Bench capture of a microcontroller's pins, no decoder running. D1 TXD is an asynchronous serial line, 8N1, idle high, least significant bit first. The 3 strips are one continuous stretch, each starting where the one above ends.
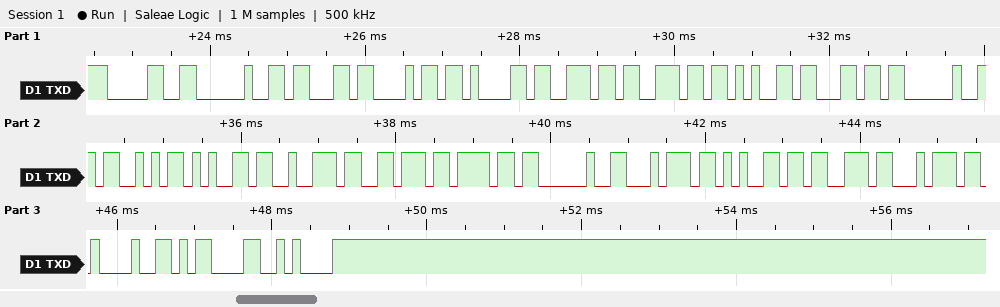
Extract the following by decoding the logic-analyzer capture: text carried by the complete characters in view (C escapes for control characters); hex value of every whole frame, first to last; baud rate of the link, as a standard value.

"0 channel Servo test!\r\n"
30 20 63 68 61 6E 6E 65 6C 20 53 65 72 76 6F 20 74 65 73 74 21 0D 0A
9600 baud
